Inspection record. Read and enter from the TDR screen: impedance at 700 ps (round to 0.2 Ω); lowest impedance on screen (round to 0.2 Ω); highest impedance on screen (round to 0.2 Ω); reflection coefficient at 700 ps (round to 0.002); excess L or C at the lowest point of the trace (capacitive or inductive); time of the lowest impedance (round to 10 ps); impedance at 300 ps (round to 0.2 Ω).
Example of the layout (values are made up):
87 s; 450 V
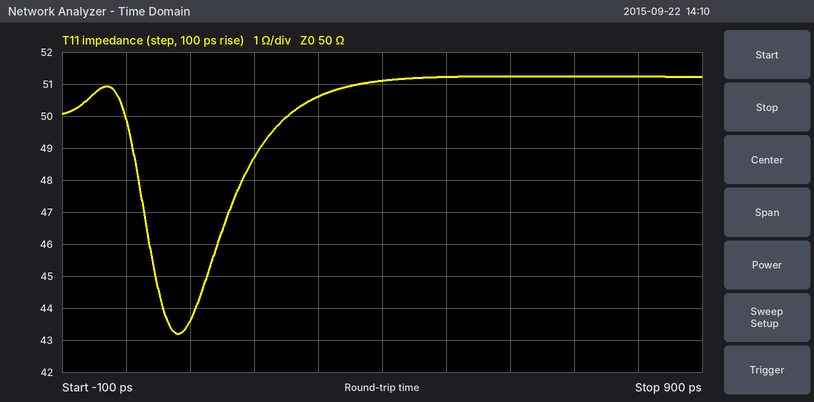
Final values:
51.2 Ω; 43.2 Ω; 51.2 Ω; +0.012; capacitive; 80 ps; 50.6 Ω
